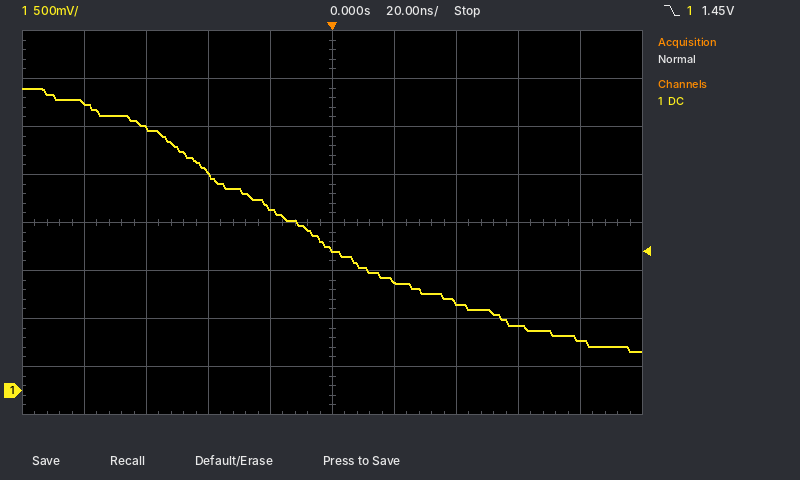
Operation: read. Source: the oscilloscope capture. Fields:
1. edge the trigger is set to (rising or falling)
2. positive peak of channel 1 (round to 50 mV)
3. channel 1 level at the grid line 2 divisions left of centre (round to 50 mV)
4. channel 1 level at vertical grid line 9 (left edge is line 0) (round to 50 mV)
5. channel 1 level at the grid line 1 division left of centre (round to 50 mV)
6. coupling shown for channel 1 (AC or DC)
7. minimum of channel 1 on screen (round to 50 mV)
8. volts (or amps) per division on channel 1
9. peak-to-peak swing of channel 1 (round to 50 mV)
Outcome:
falling
3.15 V
2.25 V
500 mV
1.90 V
DC
400 mV
500 mV
2.75 V
